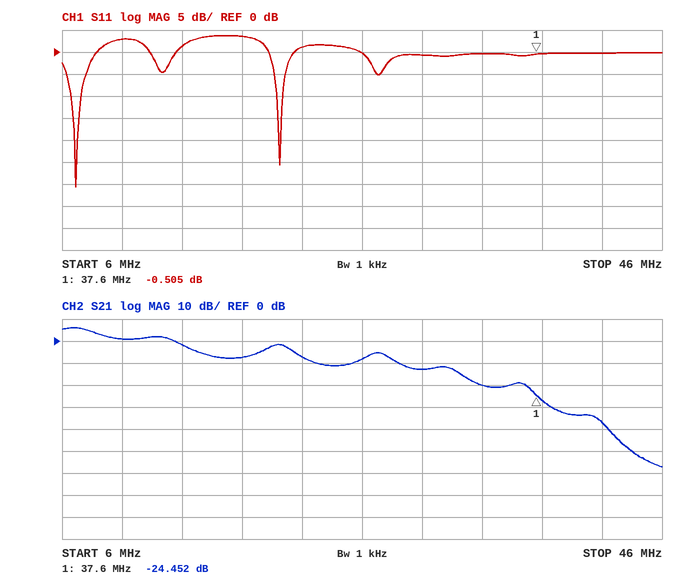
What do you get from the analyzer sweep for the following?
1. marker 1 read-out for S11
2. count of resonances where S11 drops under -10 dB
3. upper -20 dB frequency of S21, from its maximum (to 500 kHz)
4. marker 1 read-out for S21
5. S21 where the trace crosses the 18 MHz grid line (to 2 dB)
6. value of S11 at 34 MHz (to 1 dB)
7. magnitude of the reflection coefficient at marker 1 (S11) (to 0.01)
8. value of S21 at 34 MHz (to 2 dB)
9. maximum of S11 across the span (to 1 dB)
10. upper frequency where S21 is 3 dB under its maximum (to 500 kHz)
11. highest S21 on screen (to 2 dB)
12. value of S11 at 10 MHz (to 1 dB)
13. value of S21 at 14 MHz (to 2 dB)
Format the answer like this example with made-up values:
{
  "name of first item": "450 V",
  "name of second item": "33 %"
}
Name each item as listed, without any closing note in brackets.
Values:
{
  "marker 1 read-out for S11": "-0.505 dB",
  "count of resonances where S11 drops under -10 dB": "2",
  "upper -20 dB frequency of S21, from its maximum": "32.5 MHz",
  "marker 1 read-out for S21": "-24.452 dB",
  "S21 where the trace crosses the 18 MHz grid line": "-8 dB",
  "value of S11 at 34 MHz": "0 dB",
  "magnitude of the reflection coefficient at marker 1 (S11)": "0.94",
  "value of S21 at 34 MHz": "-20 dB",
  "maximum of S11 across the span": "4 dB",
  "upper frequency where S21 is 3 dB under its maximum": "8.5 MHz",
  "highest S21 on screen": "6 dB",
  "value of S11 at 10 MHz": "3 dB",
  "value of S21 at 14 MHz": "-2 dB"
}
